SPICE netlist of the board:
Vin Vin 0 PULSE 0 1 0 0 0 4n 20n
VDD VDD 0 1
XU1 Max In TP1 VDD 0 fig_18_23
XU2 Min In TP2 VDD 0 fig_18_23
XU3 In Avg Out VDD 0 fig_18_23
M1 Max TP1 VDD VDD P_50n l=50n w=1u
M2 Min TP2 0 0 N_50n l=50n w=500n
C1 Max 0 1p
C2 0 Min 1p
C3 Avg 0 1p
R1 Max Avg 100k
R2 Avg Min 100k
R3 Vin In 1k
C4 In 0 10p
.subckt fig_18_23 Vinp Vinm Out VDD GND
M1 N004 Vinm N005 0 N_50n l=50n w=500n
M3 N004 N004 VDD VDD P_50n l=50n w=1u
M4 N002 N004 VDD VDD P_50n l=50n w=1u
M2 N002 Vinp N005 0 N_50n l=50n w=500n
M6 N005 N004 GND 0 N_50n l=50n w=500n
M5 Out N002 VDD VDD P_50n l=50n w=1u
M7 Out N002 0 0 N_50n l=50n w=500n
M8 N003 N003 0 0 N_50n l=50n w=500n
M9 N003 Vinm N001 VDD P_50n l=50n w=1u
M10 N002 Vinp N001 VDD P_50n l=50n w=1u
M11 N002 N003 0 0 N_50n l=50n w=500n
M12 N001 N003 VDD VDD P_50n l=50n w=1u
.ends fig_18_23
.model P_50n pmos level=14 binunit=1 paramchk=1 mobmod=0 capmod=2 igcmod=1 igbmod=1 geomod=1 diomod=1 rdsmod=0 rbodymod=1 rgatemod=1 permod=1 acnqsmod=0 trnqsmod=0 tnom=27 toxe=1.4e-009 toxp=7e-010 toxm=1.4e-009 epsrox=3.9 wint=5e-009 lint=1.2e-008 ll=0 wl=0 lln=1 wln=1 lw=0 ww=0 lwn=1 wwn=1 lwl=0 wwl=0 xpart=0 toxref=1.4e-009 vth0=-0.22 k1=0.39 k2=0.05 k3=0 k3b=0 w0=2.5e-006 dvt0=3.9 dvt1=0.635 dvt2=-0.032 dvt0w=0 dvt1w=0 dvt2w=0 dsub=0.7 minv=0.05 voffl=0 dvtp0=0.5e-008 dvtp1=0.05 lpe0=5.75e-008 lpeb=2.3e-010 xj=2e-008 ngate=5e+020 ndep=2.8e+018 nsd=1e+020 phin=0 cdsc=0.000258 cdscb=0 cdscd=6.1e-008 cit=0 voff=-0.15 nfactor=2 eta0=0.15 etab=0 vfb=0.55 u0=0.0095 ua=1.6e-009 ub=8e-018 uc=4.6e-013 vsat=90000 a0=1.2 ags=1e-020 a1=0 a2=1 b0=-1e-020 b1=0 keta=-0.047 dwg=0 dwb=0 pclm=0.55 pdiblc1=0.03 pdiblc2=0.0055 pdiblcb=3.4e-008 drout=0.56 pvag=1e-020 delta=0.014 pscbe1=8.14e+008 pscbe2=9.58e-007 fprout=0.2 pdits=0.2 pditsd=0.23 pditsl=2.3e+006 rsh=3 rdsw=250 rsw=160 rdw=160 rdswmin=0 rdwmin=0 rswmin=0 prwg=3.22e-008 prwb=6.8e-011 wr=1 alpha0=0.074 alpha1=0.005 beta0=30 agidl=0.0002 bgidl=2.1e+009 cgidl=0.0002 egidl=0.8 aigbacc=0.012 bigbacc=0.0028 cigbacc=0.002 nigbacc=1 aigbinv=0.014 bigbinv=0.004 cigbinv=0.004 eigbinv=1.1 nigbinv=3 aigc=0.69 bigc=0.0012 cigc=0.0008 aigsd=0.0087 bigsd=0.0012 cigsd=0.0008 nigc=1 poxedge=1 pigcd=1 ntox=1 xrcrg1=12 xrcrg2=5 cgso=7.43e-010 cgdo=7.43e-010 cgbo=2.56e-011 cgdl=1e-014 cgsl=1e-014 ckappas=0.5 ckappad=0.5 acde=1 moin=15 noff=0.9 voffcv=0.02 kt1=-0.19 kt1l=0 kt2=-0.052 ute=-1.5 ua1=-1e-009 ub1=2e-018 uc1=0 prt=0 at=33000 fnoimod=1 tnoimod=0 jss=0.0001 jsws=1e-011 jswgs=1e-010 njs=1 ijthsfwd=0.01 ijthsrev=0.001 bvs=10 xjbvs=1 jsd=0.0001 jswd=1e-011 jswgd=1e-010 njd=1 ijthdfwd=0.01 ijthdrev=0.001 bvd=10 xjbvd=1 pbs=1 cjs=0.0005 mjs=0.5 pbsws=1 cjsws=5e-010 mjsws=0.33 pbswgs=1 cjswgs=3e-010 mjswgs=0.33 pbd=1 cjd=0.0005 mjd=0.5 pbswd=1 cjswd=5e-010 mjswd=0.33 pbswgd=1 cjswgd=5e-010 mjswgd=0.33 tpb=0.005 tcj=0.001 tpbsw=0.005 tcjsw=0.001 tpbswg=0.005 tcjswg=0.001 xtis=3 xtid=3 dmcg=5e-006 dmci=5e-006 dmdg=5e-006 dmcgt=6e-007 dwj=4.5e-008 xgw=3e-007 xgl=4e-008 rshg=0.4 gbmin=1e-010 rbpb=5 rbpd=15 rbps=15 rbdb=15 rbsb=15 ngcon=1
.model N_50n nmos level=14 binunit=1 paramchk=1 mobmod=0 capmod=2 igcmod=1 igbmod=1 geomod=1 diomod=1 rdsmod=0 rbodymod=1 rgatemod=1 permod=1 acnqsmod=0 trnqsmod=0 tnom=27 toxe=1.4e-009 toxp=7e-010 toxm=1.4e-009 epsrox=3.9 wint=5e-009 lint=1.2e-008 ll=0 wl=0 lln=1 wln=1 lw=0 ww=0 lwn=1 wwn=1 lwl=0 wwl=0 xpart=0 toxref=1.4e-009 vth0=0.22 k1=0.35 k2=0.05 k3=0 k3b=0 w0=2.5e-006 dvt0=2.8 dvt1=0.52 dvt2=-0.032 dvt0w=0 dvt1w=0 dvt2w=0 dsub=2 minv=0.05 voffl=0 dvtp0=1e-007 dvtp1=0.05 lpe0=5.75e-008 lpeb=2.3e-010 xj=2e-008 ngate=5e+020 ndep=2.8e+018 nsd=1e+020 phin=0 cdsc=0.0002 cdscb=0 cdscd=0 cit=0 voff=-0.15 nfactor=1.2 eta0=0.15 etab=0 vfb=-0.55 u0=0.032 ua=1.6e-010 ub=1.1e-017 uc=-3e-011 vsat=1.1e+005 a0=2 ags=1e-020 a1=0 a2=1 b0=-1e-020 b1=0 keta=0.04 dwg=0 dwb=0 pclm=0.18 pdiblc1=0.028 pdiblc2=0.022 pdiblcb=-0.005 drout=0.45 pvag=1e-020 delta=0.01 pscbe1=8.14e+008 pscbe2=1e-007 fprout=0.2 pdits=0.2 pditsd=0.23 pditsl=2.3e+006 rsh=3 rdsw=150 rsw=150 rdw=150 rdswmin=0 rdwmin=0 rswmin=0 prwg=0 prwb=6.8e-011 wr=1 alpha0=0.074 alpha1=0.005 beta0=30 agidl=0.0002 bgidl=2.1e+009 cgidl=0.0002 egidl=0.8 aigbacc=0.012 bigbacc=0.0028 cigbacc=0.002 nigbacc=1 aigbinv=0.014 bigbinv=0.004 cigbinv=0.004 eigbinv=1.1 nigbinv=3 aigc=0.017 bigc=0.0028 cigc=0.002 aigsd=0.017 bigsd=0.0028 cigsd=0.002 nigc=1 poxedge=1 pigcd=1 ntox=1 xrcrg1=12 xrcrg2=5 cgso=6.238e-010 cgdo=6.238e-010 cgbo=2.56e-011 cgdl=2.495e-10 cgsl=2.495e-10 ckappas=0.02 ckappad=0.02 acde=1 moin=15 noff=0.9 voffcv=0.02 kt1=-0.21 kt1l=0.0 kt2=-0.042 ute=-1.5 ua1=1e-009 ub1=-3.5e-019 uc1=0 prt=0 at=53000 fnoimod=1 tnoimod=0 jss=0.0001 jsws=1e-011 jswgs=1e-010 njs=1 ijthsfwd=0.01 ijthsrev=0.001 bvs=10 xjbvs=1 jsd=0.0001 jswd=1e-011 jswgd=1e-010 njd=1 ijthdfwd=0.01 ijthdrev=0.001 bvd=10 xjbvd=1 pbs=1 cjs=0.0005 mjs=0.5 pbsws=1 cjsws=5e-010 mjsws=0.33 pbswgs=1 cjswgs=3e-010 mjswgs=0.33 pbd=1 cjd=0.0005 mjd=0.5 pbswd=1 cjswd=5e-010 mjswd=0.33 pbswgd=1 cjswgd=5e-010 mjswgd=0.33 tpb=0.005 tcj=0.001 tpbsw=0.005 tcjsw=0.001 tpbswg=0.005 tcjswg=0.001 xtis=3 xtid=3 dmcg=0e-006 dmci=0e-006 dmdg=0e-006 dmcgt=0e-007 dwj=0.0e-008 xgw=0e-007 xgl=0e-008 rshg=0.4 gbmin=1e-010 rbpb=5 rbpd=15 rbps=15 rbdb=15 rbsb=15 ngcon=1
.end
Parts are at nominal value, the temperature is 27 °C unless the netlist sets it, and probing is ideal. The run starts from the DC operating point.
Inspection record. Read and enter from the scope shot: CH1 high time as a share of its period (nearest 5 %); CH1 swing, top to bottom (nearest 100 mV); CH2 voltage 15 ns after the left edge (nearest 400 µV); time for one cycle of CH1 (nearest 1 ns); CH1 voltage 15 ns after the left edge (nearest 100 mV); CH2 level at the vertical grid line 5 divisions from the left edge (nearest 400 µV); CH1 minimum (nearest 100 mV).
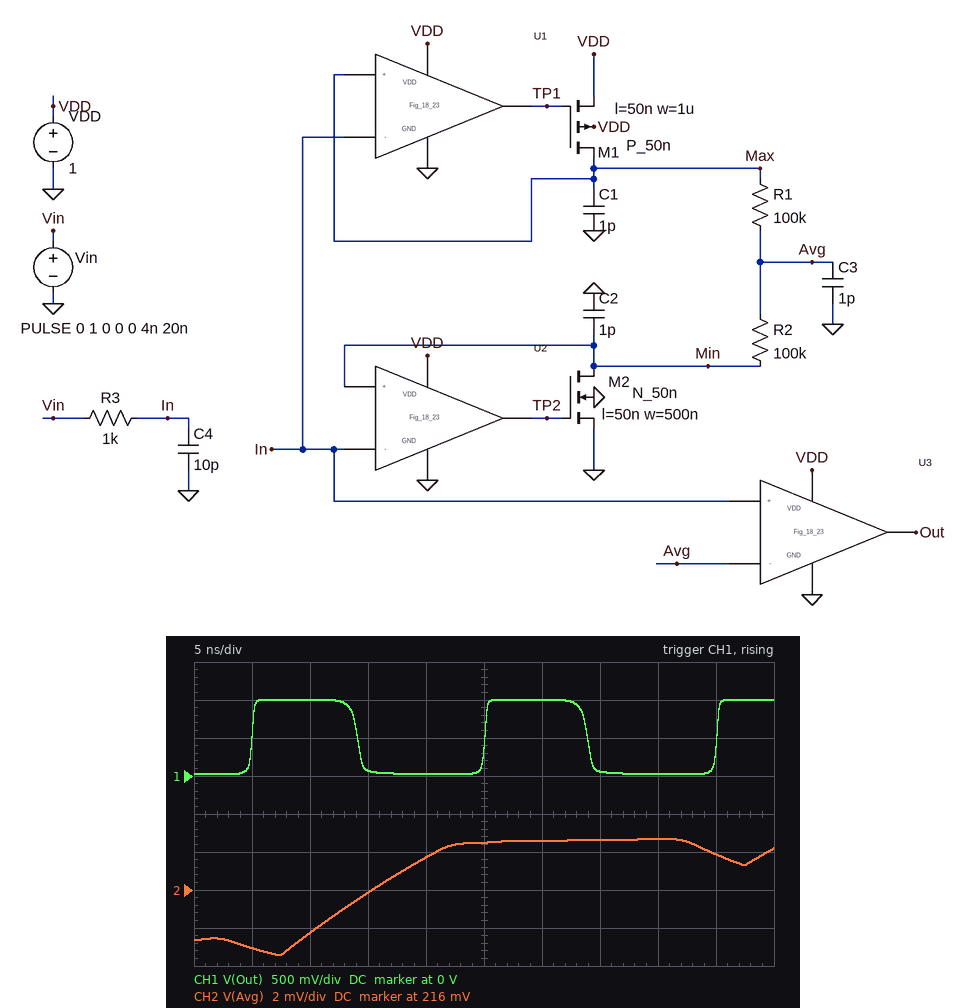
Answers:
45 %
1.0 V
216.0 mV
20 ns
100 mV
218.4 mV
0 V
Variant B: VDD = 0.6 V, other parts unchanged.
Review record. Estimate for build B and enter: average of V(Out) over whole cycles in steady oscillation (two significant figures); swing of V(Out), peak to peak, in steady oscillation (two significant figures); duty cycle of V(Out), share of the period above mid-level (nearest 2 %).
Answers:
290 mV
600 mV
48 %
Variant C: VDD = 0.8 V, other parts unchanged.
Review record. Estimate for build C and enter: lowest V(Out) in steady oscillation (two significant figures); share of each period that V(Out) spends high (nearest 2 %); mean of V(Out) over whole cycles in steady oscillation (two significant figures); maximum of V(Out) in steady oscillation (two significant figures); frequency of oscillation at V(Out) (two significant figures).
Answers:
1.1 mV
42 %
340 mV
800 mV
50 MHz
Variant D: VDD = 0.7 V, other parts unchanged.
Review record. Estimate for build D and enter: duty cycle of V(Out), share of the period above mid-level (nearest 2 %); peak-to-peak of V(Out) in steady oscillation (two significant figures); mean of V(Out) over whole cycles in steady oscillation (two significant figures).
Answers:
44 %
700 mV
310 mV
